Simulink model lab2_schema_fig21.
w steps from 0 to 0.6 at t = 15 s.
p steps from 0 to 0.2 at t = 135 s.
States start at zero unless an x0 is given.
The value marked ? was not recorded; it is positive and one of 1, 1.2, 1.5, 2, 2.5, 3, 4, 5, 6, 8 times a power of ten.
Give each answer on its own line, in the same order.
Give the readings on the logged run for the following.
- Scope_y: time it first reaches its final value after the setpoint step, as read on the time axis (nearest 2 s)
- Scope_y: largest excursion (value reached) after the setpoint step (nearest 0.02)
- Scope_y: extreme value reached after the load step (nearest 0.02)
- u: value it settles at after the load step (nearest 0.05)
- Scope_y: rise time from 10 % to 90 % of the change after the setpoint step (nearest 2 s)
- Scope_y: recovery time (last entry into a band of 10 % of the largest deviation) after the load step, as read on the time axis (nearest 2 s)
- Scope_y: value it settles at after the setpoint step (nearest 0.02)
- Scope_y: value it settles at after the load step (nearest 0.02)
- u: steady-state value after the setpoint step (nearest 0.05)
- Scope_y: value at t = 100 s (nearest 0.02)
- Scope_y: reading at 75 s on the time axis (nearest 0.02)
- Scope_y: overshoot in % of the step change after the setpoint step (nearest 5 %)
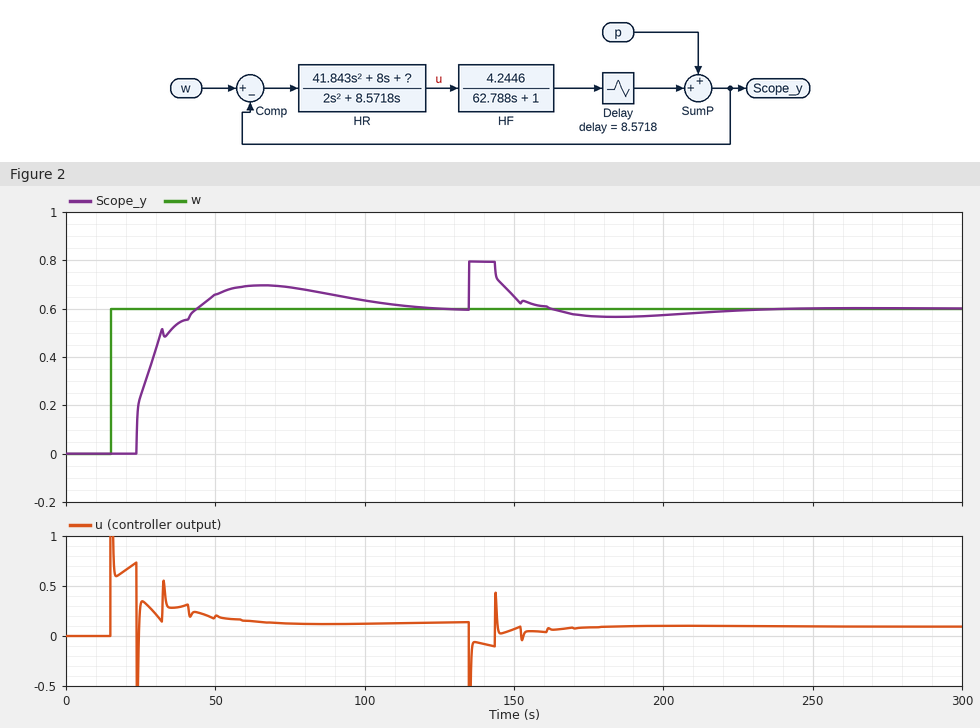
44 s
0.70
0.80
0.10
14 s
208 s
0.60
0.60
0.15
0.64
0.68
15 %
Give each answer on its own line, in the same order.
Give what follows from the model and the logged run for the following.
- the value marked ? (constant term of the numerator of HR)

0.3
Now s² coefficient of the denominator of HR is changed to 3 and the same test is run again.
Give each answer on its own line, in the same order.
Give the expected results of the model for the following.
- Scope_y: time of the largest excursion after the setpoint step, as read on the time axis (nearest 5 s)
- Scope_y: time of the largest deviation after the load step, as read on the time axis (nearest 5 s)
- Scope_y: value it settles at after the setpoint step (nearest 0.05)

65 s
135 s
0.60
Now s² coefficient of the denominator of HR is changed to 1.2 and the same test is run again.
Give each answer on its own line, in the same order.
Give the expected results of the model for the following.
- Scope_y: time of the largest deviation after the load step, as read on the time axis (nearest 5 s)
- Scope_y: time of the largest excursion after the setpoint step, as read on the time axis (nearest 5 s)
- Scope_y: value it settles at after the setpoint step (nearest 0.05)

135 s
65 s
0.60
